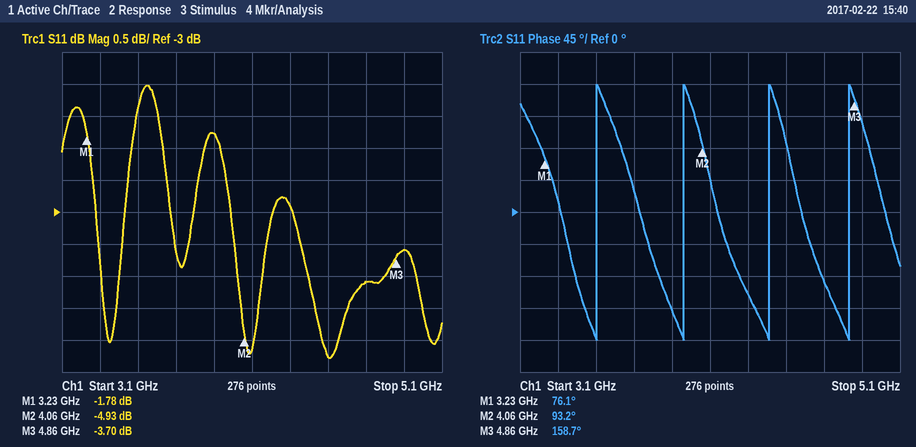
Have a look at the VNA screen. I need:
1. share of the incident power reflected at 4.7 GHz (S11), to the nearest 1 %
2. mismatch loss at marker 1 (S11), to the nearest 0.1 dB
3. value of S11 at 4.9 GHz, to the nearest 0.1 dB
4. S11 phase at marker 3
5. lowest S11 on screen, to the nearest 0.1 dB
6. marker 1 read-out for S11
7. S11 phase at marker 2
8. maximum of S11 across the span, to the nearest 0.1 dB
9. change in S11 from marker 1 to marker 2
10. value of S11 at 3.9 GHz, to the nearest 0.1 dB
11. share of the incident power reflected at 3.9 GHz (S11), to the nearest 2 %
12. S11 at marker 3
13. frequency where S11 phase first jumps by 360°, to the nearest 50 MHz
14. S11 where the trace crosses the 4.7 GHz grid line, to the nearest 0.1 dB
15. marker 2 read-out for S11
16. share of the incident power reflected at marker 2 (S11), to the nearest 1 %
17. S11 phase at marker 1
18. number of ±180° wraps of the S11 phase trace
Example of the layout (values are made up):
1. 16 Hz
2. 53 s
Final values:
1. 39 %
2. 4.7 dB
3. -3.6 dB
4. 158.7°
5. -5.3 dB
6. -1.78 dB
7. 93.2°
8. -1.0 dB
9. -3.15 dB
10. -1.8 dB
11. 66 %
12. -3.70 dB
13. 3.50 GHz
14. -4.1 dB
15. -4.93 dB
16. 32 %
17. 76.1°
18. 4
